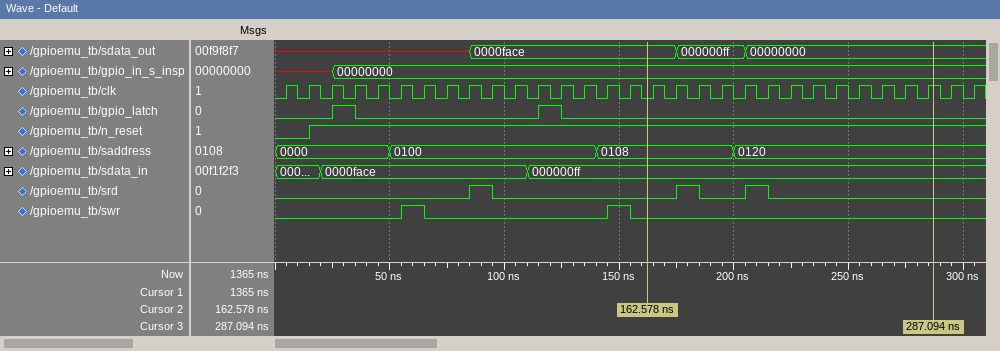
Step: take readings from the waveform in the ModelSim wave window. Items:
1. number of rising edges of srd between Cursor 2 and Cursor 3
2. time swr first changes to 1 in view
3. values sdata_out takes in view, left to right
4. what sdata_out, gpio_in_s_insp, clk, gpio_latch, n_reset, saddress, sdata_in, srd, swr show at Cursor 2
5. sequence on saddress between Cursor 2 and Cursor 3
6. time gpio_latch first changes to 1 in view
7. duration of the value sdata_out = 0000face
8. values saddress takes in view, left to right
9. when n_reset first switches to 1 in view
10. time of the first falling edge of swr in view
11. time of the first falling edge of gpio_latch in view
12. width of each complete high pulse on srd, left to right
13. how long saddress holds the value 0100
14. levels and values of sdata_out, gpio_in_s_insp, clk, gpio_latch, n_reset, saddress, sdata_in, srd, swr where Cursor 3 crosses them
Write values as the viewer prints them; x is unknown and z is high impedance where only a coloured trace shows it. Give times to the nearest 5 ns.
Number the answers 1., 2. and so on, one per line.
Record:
1. 2
2. 55 ns
3. x, 0000face, 000000ff, 00000000
4. sdata_out=0000face, gpio_in_s_insp=00000000, clk=0, gpio_latch=0, n_reset=1, saddress=0108, sdata_in=000000ff, srd=0, swr=0
5. 0108, 0120
6. 25 ns
7. 90 ns
8. 0000, 0100, 0108, 0120
9. 15 ns
10. 65 ns
11. 35 ns
12. 10 ns, 10 ns, 10 ns
13. 90 ns
14. sdata_out=00000000, gpio_in_s_insp=00000000, clk=1, gpio_latch=0, n_reset=1, saddress=0120, sdata_in=000000ff, srd=0, swr=0
